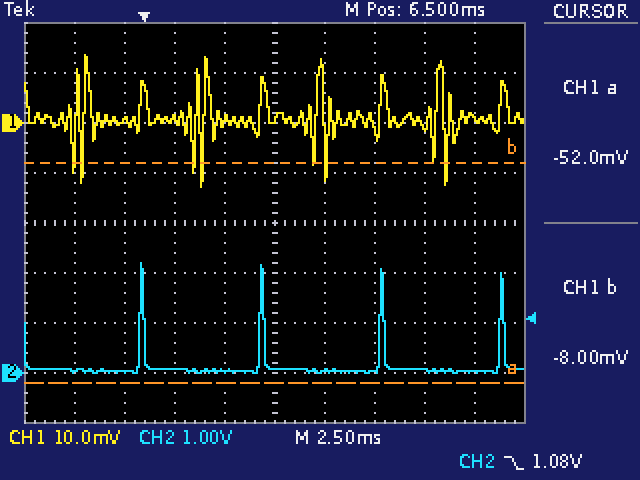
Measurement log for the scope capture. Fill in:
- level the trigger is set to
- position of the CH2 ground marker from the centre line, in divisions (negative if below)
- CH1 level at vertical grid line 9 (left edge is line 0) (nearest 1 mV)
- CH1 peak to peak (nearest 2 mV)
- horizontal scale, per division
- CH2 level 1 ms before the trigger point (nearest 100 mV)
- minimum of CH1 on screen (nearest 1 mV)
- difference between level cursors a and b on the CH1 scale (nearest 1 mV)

1.08 V
-3.0 div
1 mV
26 mV
2.5 ms
0.0 V
-13 mV
44 mV
